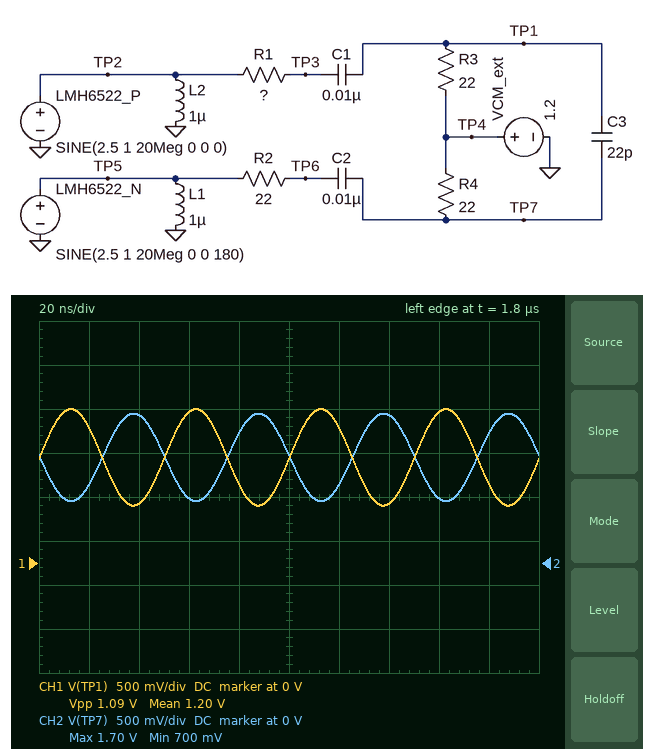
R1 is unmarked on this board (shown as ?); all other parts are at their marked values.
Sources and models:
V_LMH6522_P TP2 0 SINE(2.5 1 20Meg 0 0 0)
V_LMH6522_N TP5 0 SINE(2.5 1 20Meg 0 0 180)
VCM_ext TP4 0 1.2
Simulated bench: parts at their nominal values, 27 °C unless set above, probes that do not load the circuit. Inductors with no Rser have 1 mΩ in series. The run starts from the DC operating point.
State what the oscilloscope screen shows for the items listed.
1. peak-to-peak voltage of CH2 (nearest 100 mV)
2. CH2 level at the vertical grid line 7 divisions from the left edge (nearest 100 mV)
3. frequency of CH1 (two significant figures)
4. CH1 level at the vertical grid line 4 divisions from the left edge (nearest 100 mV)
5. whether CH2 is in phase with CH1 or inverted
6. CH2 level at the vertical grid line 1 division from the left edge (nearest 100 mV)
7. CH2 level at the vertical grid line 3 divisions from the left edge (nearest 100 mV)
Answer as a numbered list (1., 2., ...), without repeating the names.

1. 1.0 V
2. 1.7 V
3. 20 MHz
4. 900 mV
5. inverted
6. 900 mV
7. 700 mV
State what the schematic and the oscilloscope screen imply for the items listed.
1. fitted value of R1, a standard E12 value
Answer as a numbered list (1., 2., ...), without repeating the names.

1. 18 Ω
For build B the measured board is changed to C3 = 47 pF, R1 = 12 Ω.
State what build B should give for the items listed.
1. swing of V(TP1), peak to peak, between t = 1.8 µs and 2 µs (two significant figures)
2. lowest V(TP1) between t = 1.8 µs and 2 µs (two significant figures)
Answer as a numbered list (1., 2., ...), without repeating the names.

1. 1.3 V
2. 560 mV
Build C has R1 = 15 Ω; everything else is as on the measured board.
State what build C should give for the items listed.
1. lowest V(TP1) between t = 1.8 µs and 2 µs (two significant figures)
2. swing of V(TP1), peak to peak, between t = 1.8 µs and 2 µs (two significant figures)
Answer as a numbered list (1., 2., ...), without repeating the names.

1. 610 mV
2. 1.2 V
